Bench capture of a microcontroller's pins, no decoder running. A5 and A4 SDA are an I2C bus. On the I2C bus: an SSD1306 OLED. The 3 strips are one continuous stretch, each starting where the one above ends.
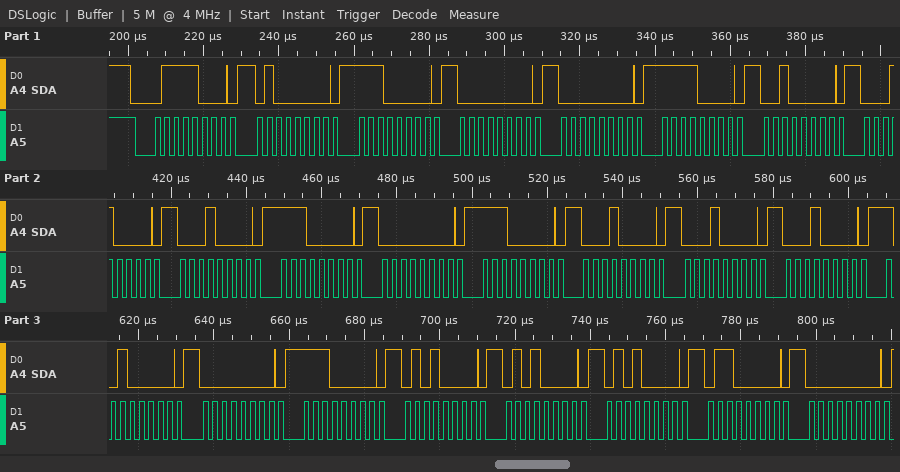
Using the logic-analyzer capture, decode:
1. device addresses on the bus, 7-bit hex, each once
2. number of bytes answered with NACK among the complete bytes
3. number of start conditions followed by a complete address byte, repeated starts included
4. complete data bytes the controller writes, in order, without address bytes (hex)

0x3C
0
1
40 E0 00 00 F0 20 10 10 E0 00 E0 10 10 10 A0 00 E0 50 50 50 60 00
